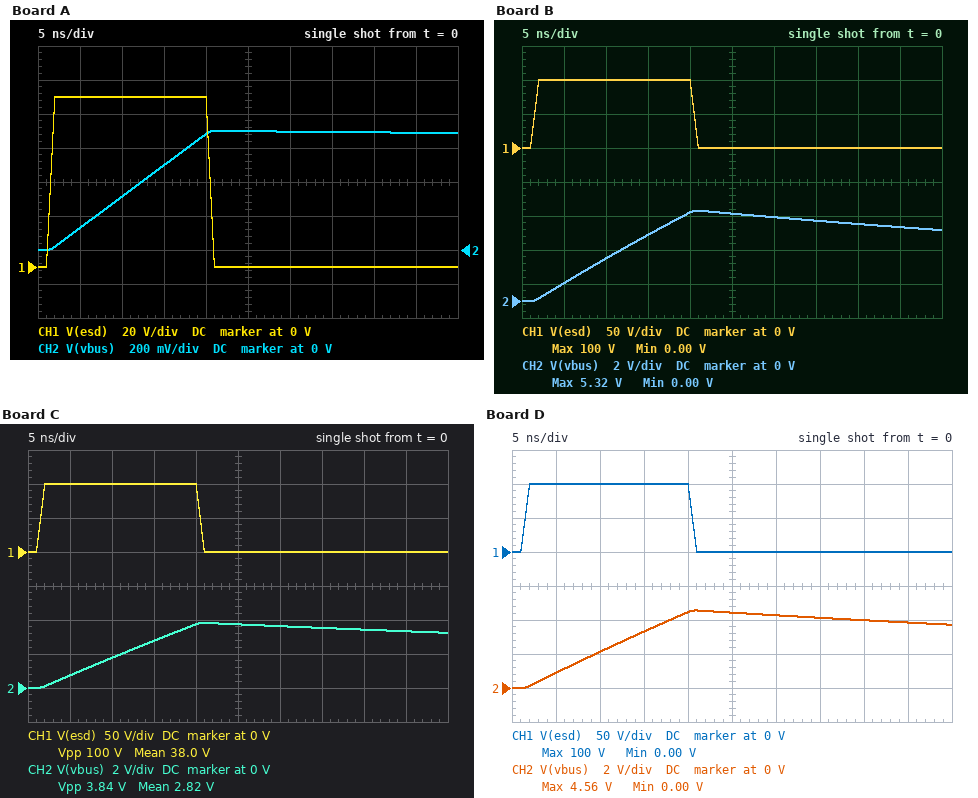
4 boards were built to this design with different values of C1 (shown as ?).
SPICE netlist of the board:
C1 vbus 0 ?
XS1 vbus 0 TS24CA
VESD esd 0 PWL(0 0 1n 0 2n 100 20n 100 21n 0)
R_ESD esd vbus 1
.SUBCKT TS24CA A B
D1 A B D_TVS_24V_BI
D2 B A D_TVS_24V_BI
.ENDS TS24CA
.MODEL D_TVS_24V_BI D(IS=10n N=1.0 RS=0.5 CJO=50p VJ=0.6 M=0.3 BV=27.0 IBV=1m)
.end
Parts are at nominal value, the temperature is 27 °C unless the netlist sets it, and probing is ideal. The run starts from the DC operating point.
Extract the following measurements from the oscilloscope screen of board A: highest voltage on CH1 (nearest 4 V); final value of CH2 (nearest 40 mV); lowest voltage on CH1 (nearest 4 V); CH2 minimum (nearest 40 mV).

100 V
680 mV
0 V
0 V
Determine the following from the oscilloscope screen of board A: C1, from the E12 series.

2.7 µF
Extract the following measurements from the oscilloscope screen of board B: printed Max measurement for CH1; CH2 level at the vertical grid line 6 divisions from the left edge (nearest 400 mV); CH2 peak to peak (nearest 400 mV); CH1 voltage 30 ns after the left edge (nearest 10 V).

100 V
4.8 V
5.2 V
0 V
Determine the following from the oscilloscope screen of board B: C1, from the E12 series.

330 nF
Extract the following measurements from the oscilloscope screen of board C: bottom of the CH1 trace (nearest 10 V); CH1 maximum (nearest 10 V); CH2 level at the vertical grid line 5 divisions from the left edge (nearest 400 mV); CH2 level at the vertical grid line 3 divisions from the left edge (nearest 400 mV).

0 V
100 V
3.6 V
2.8 V
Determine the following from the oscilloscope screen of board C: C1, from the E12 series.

470 nF
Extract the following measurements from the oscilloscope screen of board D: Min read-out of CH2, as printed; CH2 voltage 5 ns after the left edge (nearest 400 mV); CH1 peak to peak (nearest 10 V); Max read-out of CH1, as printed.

0.00 V
800 mV
100 V
100 V
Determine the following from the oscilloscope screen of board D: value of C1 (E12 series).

390 nF
